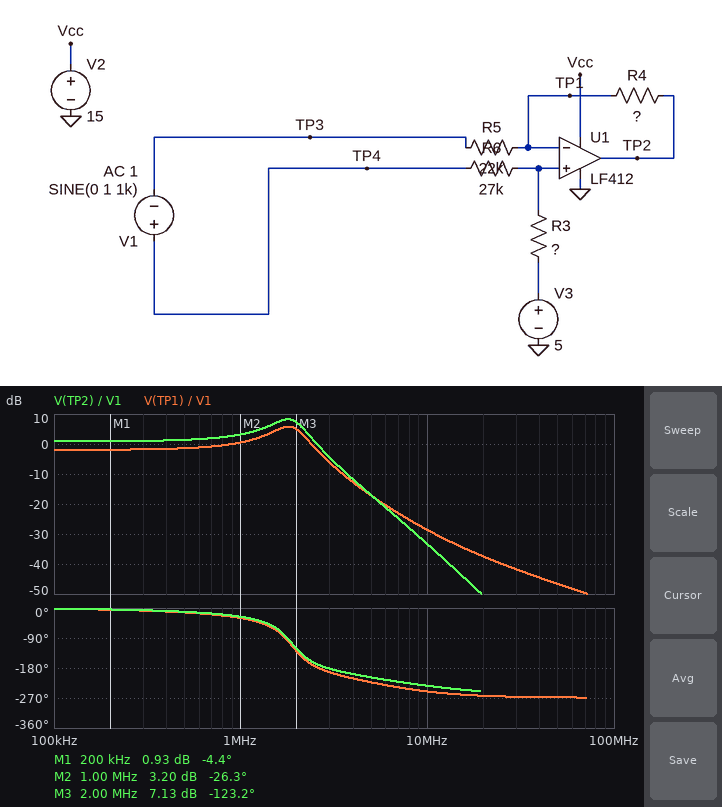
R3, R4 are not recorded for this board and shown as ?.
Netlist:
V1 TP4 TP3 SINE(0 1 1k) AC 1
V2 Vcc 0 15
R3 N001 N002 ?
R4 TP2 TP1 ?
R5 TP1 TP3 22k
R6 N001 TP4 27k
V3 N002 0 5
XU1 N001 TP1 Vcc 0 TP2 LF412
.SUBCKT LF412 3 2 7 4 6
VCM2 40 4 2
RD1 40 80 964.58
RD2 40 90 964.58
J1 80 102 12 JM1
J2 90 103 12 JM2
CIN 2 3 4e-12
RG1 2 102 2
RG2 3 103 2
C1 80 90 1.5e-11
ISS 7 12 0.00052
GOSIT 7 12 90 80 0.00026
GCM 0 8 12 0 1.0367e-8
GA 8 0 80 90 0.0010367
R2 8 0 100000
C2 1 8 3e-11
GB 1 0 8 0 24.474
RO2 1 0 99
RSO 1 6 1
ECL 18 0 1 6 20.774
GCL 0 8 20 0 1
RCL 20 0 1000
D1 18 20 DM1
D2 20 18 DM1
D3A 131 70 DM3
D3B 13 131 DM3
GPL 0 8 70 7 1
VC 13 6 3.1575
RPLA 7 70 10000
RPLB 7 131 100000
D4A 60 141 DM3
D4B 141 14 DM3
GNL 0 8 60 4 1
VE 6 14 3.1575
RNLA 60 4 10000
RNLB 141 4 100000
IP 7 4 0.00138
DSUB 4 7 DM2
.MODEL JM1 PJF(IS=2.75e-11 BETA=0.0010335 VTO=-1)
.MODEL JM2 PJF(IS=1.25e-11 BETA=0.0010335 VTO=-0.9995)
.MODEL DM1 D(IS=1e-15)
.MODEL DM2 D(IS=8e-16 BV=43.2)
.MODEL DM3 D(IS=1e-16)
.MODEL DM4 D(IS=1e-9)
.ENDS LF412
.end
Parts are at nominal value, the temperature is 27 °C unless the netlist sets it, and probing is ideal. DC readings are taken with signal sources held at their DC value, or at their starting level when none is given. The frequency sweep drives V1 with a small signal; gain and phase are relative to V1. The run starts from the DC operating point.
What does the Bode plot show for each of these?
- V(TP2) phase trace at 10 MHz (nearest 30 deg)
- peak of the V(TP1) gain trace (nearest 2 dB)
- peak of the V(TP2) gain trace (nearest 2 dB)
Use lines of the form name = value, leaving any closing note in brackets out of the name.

V(TP2) phase trace at 10 MHz = -240 deg
peak of the V(TP1) gain trace = 6 dB
peak of the V(TP2) gain trace = 8 dB
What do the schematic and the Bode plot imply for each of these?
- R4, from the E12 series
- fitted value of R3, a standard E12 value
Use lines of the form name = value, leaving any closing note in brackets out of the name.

R4, from the E12 series = 15 kΩ
fitted value of R3, a standard E12 value = 39 kΩ
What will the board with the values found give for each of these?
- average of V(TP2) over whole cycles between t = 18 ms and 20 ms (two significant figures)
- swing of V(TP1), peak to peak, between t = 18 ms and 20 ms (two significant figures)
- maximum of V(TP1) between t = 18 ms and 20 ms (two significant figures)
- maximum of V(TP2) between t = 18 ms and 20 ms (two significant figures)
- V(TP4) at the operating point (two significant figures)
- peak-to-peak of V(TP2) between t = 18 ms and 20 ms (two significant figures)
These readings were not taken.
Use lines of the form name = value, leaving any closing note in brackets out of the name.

average of V(TP2) over whole cycles between t = 18 ms and 20 ms = 5.0 V
swing of V(TP1), peak to peak, between t = 18 ms and 20 ms = 1.6 V
maximum of V(TP1) between t = 18 ms and 20 ms = 5.8 V
maximum of V(TP2) between t = 18 ms and 20 ms = 6.1 V
V(TP4) at the operating point = 5.0 V
peak-to-peak of V(TP2) between t = 18 ms and 20 ms = 2.2 V
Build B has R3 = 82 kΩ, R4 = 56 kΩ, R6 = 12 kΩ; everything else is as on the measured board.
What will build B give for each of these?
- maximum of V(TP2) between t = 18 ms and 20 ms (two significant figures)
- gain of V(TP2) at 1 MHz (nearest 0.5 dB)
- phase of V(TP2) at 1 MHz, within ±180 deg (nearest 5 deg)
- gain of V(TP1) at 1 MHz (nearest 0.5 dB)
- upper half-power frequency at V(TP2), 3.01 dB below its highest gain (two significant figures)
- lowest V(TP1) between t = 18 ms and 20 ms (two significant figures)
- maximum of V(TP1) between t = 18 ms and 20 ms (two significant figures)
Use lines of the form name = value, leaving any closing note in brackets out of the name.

maximum of V(TP2) between t = 18 ms and 20 ms = 9.1 V
gain of V(TP2) at 1 MHz = 14.0 dB
phase of V(TP2) at 1 MHz, within ±180 deg = -75 deg
gain of V(TP1) at 1 MHz = 9.5 dB
upper half-power frequency at V(TP2), 3.01 dB below its highest gain = 1.4 MHz
lowest V(TP1) between t = 18 ms and 20 ms = 3.3 V
maximum of V(TP1) between t = 18 ms and 20 ms = 7.4 V
